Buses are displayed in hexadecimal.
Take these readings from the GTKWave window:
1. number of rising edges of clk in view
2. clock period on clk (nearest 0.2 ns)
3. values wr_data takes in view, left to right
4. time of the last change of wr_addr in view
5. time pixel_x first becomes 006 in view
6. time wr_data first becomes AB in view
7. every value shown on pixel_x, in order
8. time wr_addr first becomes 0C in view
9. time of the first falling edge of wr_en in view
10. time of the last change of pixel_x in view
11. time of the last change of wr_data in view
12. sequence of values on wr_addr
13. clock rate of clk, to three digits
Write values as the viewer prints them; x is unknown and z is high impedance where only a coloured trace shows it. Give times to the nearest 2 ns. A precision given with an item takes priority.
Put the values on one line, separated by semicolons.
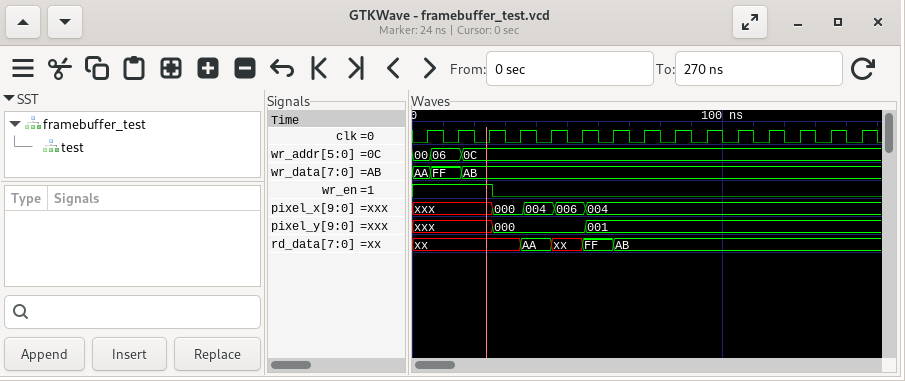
15; 10 ns; AA, FF, AB; 16 ns; 46 ns; 16 ns; xxx, 000, 004, 006, 004; 16 ns; 26 ns; 56 ns; 16 ns; 00, 06, 0C; 100 MHz
